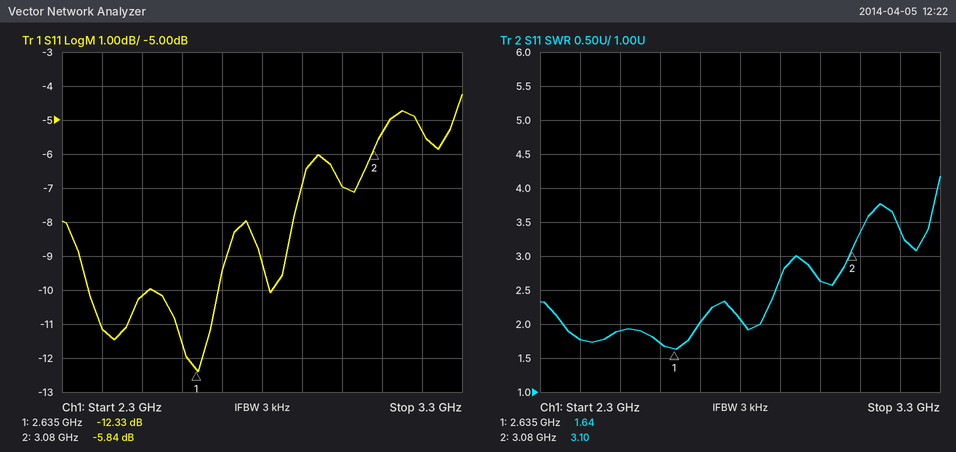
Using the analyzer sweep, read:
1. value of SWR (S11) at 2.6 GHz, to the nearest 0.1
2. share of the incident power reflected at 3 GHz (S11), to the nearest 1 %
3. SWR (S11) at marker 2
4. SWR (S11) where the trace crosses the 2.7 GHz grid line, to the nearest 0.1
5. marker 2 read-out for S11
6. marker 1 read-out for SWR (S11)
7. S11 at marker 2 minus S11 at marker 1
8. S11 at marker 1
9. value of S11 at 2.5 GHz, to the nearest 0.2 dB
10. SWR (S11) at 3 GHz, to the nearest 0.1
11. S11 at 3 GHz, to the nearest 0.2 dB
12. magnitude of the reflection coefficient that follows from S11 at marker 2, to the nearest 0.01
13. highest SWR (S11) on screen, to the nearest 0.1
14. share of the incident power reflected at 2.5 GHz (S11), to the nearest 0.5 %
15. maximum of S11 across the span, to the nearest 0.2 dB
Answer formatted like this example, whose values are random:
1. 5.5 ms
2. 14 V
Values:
1. 1.7
2. 20 %
3. 3.10
4. 2.0
5. -5.84 dB
6. 1.64
7. 6.49 dB
8. -12.33 dB
9. -10.2 dB
10. 2.6
11. -7.0 dB
12. 0.51
13. 4.2
14. 9.5 %
15. -4.2 dB
